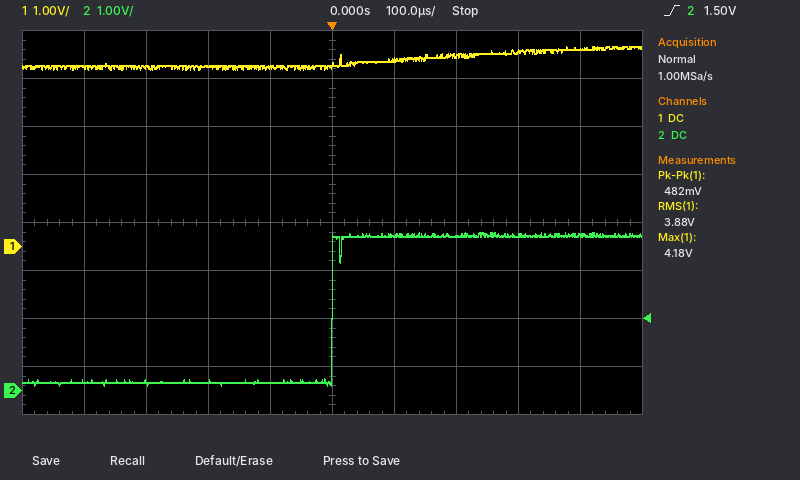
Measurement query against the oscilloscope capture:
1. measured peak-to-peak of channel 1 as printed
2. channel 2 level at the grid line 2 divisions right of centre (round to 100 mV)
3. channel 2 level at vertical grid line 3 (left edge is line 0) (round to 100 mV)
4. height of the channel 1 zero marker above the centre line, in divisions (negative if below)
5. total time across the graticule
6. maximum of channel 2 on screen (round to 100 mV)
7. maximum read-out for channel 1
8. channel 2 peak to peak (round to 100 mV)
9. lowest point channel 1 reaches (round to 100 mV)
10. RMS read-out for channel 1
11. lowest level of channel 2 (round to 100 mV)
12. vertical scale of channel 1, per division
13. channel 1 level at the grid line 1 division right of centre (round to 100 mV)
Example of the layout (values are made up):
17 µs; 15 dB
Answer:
482 mV; 3.2 V; 200 mV; -0.5 div; 1 ms; 3.3 V; 4.18 V; 3.2 V; 3.7 V; 3.88 V; 100 mV; 1 V; 3.9 V
